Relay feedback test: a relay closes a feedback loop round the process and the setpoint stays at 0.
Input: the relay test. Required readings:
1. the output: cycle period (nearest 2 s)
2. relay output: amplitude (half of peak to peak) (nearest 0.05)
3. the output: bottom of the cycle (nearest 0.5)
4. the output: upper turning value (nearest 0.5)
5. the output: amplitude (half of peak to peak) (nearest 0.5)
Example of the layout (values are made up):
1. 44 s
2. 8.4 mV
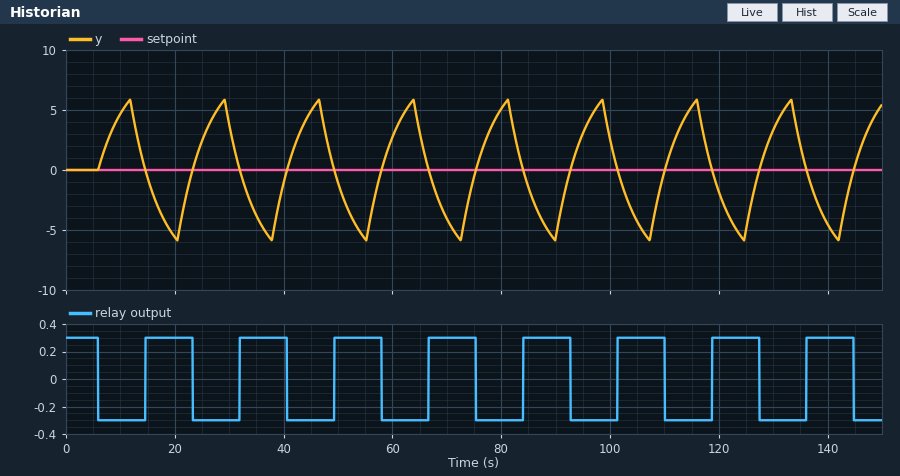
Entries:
1. 18 s
2. 0.30
3. -6.0
4. 6.0
5. 6.0
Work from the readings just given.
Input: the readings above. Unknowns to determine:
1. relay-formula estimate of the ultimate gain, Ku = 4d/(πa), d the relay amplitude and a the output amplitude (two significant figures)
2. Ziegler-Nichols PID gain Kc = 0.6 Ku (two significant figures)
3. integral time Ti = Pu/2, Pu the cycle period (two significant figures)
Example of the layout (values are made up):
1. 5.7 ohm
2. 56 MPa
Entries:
1. 0.064
2. 0.038
3. 9.0 s
